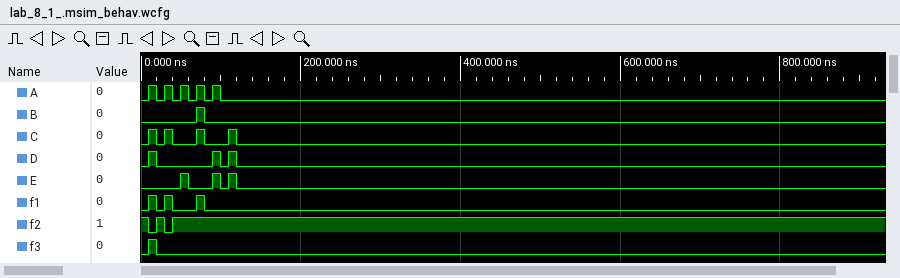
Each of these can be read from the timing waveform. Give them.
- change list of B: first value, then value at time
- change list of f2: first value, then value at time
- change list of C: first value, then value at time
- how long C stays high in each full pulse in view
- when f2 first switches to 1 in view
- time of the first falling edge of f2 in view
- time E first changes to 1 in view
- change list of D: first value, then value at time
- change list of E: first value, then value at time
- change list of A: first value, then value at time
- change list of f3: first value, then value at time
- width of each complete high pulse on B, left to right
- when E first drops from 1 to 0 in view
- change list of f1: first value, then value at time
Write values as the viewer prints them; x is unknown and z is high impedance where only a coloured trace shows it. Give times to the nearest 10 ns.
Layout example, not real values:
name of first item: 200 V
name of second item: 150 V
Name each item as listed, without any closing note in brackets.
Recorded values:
change list of B: first value, then value at time: 0, 1 at 70 ns, 0 at 80 ns
change list of f2: first value, then value at time: 1, 0 at 10 ns, 1 at 20 ns, 0 at 30 ns, 1 at 40 ns
change list of C: first value, then value at time: 0, 1 at 10 ns, 0 at 20 ns, 1 at 30 ns, 0 at 40 ns, 1 at 70 ns, 0 at 80 ns, 1 at 110 ns, 0 at 120 ns
how long C stays high in each full pulse in view: 10 ns, 10 ns, 10 ns, 10 ns
when f2 first switches to 1 in view: 20 ns
time of the first falling edge of f2 in view: 10 ns
time E first changes to 1 in view: 50 ns
change list of D: first value, then value at time: 0, 1 at 10 ns, 0 at 20 ns, 1 at 90 ns, 0 at 100 ns, 1 at 110 ns, 0 at 120 ns
change list of E: first value, then value at time: 0, 1 at 50 ns, 0 at 60 ns, 1 at 90 ns, 0 at 100 ns, 1 at 110 ns, 0 at 120 ns
change list of A: first value, then value at time: 0, 1 at 10 ns, 0 at 20 ns, 1 at 30 ns, 0 at 40 ns, 1 at 50 ns, 0 at 60 ns, 1 at 70 ns, 0 at 80 ns, 1 at 90 ns, 0 at 100 ns
change list of f3: first value, then value at time: 0, 1 at 10 ns, 0 at 20 ns
width of each complete high pulse on B, left to right: 10 ns
when E first drops from 1 to 0 in view: 60 ns
change list of f1: first value, then value at time: 0, 1 at 10 ns, 0 at 20 ns, 1 at 30 ns, 0 at 40 ns, 1 at 70 ns, 0 at 80 ns
